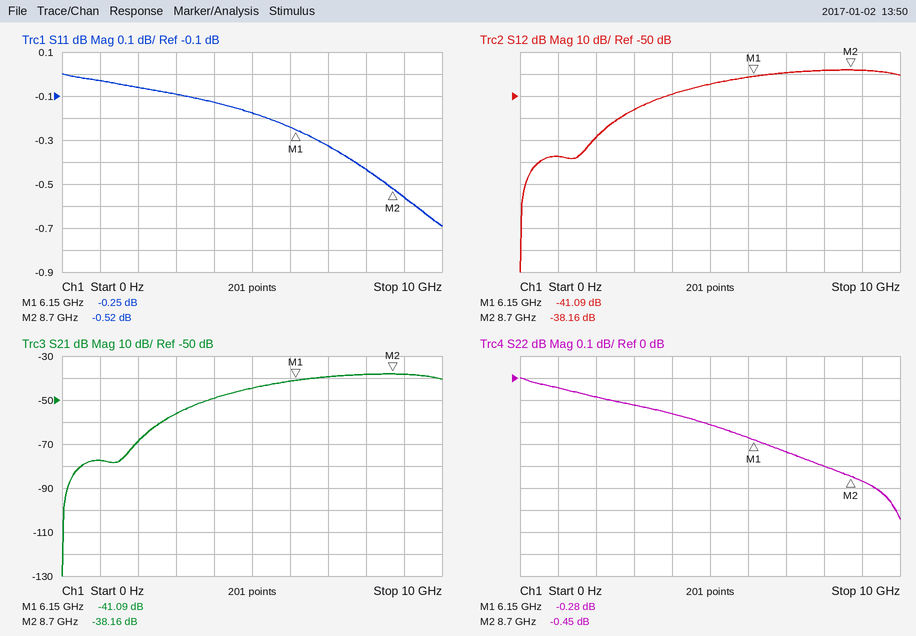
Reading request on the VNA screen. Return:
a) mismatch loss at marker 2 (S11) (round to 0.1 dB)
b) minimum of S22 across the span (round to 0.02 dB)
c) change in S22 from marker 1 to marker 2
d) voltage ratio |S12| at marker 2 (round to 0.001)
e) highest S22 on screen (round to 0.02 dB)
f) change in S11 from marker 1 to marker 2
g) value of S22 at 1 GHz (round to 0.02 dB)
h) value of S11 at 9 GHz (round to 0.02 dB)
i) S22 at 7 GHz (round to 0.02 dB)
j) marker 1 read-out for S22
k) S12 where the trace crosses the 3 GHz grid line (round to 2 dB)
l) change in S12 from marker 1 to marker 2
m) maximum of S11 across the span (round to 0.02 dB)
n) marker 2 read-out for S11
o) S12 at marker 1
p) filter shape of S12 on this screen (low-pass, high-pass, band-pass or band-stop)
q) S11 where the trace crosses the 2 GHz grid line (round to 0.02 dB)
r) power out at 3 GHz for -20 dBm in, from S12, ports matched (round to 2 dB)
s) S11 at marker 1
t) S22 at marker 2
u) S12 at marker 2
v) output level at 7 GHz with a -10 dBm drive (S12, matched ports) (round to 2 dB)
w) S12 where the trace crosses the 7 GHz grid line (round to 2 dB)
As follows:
9.5 dB
-0.64 dB
-0.17 dB
0.012
0.00 dB
-0.27 dB
-0.04 dB
-0.56 dB
-0.34 dB
-0.28 dB
-56 dB
2.93 dB
0.00 dB
-0.52 dB
-41.09 dB
high-pass
-0.06 dB
-76 dBm
-0.25 dB
-0.45 dB
-38.16 dB
-50 dBm
-40 dB
